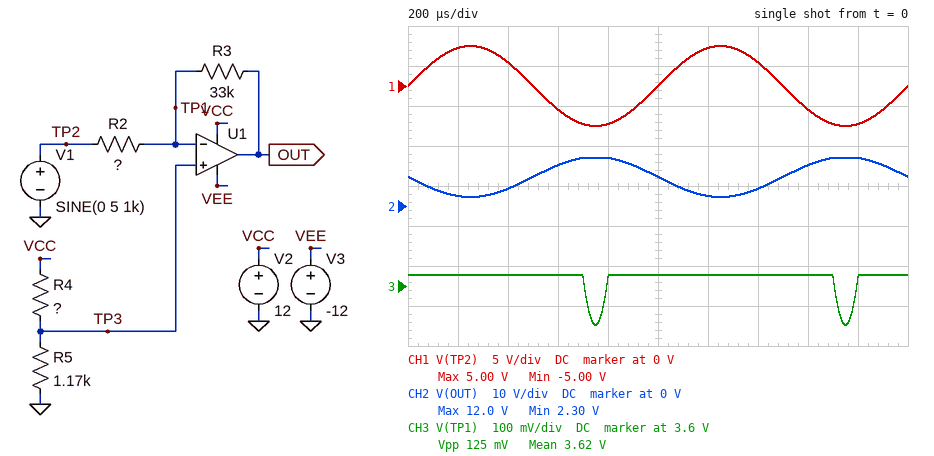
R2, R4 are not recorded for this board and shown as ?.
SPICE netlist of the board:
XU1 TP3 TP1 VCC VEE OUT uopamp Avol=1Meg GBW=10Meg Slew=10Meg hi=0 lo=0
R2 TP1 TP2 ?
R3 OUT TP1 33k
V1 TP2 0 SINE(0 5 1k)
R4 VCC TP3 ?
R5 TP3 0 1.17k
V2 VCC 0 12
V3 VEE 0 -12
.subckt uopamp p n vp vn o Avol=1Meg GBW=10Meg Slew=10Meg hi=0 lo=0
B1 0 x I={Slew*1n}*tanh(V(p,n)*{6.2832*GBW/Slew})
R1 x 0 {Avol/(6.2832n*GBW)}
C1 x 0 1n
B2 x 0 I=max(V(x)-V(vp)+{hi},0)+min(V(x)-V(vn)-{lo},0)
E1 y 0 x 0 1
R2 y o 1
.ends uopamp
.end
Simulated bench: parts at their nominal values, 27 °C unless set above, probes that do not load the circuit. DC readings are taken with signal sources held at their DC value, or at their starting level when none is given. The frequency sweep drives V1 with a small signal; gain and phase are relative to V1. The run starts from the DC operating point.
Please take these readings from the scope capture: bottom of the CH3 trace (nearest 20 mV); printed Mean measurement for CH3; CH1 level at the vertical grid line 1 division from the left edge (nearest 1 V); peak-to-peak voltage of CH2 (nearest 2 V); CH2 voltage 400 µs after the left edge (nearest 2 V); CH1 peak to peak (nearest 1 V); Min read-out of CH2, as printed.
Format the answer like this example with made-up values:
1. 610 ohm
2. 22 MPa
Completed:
1. 3.50 V
2. 3.62 V
3. 5 V
4. 10 V
5. 4 V
6. 10 V
7. 2.30 V
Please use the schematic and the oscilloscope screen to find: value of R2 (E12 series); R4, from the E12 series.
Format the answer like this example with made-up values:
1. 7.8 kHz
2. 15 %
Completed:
1. 33 kΩ
2. 2.7 kΩ
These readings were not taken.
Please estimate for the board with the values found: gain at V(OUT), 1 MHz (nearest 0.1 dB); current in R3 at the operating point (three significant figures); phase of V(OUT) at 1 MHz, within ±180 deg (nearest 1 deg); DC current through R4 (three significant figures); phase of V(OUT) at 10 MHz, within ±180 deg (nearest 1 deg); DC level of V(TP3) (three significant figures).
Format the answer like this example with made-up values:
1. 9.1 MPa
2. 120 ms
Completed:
1. -0.2 dB
2. 110 µA
3. 169 deg
4. 3.10 mA
5. 117 deg
6. 3.63 V
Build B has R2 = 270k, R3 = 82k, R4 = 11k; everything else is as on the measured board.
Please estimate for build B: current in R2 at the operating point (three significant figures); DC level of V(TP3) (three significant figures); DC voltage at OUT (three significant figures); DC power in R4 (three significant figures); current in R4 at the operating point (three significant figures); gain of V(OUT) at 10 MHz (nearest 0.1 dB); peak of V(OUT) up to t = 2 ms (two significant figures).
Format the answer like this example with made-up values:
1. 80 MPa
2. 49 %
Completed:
1. 4.27 µA
2. 1.15 V
3. 1.50 V
4. 10.7 mW
5. 986 µA
6. -14.7 dB
7. 3.0 V
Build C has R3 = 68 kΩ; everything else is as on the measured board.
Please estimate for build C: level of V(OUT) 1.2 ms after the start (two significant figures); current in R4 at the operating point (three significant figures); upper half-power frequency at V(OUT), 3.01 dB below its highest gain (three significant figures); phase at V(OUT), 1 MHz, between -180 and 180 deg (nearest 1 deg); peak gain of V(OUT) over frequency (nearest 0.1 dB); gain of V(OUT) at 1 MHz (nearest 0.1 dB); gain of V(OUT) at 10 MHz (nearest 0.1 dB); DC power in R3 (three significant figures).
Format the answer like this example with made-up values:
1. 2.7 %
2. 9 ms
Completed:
1. 1.3 V
2. 3.10 mA
3. 3.27 MHz
4. 163 deg
5. 6.3 dB
6. 5.9 dB
7. -3.9 dB
8. 822 µW
